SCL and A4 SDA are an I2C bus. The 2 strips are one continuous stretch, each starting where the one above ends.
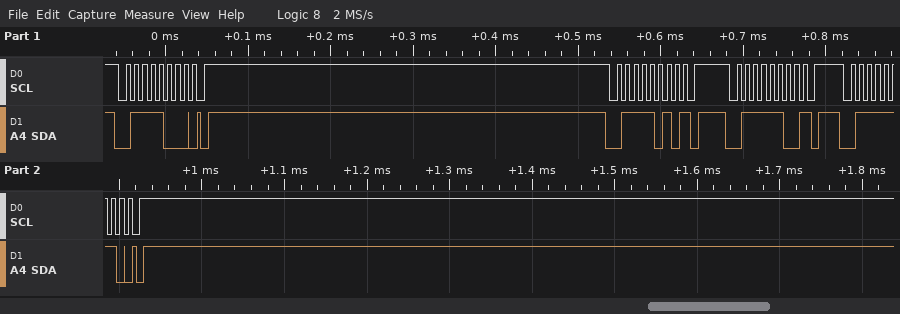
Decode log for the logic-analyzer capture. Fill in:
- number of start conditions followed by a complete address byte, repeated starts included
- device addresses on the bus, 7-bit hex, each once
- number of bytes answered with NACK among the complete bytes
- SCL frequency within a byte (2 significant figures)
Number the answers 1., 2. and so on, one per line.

1. 4
2. 0x3C 0x3D 0x3E 0x3F
3. 2
4. 100 kHz
